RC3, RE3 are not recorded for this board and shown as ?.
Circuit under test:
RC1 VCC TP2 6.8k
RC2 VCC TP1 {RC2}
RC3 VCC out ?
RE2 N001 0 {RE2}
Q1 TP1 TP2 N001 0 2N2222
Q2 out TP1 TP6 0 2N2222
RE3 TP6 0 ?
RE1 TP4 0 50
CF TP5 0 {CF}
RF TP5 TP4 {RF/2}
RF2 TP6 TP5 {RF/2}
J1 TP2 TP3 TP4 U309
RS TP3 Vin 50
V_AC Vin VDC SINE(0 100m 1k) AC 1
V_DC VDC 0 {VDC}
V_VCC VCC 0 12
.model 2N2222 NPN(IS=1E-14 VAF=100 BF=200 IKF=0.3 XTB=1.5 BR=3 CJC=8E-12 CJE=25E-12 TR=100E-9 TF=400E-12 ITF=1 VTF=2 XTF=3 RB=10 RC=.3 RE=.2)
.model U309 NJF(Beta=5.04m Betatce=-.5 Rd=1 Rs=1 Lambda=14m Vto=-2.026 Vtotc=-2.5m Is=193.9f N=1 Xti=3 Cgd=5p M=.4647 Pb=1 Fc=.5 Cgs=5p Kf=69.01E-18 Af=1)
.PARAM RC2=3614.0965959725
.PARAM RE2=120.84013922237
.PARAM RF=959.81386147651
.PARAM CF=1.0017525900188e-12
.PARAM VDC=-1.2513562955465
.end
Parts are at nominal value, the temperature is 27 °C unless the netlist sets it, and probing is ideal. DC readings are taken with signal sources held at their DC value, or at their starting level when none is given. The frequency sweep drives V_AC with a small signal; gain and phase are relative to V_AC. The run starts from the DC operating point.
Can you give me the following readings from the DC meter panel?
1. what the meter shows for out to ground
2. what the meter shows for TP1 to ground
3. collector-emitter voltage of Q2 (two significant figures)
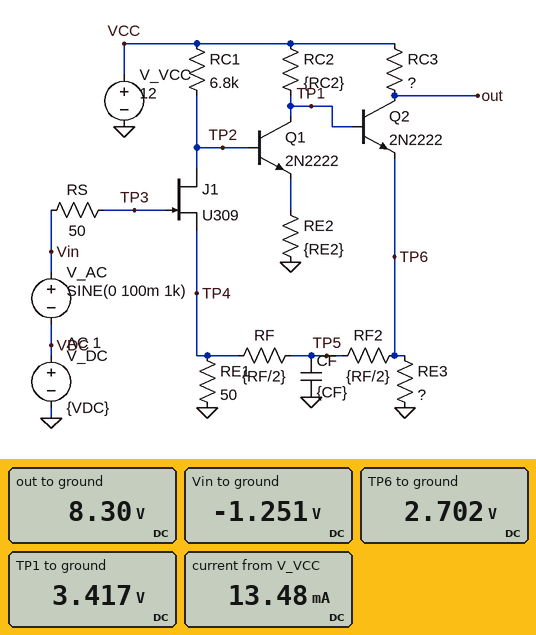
8.30 V
3.417 V
5.6 V
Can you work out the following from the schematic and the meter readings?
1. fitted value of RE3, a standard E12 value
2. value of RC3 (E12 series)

390 Ω
390 Ω
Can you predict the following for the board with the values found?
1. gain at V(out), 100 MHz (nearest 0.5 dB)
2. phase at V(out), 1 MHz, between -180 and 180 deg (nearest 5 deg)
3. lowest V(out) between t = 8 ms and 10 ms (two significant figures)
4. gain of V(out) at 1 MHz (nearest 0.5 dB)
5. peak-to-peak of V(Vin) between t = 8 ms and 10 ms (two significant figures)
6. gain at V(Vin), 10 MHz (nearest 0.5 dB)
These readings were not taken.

-2.5 dB
170 deg
5.6 V
28.5 dB
200 mV
0 dB
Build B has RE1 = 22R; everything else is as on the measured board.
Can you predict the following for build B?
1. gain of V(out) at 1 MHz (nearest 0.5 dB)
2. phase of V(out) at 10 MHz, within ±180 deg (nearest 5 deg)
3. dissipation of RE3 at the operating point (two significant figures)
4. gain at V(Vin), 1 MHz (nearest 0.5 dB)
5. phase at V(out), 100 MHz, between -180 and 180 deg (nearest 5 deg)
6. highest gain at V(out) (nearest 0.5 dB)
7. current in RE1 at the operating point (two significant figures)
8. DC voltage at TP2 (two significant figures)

-16.5 dB
-80 deg
71 mW
0 dB
170 deg
-10.5 dB
7.0 mA
550 mV
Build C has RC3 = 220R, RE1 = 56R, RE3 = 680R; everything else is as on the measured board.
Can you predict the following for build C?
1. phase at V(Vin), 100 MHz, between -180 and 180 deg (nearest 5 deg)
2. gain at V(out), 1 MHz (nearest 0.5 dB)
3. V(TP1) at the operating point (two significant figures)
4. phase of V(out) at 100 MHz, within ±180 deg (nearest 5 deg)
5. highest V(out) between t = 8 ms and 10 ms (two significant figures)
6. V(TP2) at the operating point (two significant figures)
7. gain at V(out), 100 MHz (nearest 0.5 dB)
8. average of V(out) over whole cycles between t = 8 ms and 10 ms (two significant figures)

0 deg
19.5 dB
3.0 V
-100 deg
12 V
980 mV
-6.0 dB
11 V
